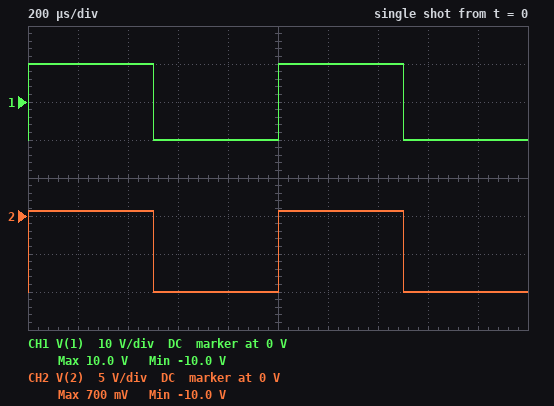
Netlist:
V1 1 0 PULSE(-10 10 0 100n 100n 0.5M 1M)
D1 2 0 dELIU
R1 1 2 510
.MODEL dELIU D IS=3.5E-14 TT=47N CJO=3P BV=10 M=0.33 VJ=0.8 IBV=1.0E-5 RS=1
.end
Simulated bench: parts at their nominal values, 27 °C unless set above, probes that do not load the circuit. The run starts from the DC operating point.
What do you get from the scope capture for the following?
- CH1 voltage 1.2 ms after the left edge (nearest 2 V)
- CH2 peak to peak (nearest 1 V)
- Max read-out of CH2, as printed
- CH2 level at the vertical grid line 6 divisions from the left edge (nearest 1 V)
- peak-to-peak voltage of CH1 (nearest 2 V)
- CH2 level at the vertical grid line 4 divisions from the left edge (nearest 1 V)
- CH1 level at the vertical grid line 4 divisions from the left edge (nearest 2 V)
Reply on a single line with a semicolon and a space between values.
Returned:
10 V; 11 V; 700 mV; 1 V; 20 V; -10 V; -10 V
